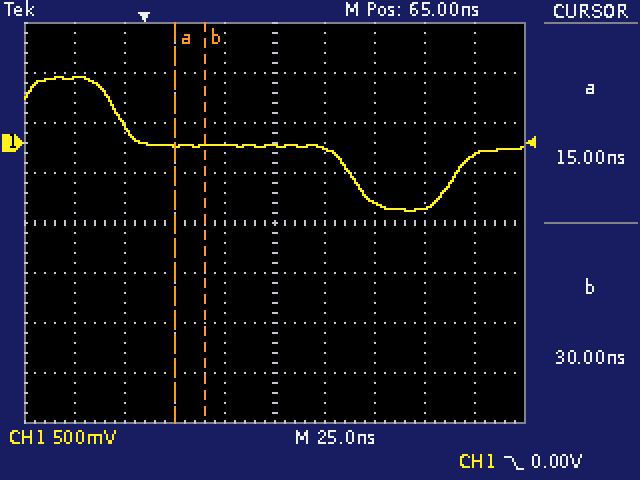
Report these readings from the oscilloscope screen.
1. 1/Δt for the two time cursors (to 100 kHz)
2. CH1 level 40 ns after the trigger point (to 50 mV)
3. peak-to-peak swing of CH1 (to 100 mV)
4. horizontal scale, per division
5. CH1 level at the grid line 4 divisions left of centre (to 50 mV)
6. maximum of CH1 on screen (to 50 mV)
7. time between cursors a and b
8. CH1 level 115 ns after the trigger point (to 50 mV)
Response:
66.7 MHz
0 mV
1.30 V
25 ns
650 mV
650 mV
15.0 ns
-600 mV
